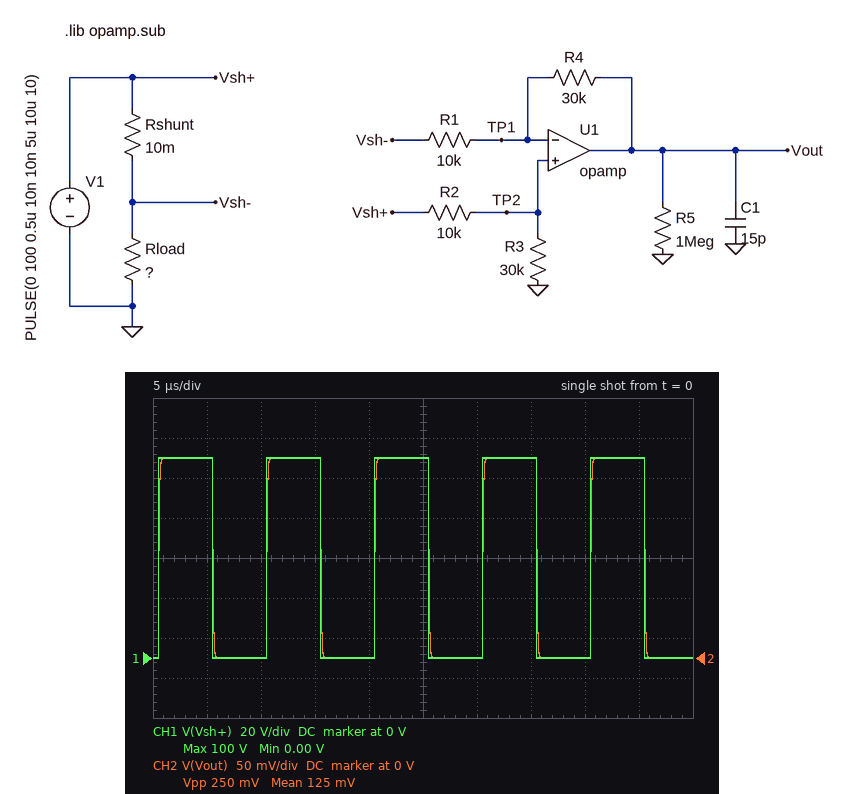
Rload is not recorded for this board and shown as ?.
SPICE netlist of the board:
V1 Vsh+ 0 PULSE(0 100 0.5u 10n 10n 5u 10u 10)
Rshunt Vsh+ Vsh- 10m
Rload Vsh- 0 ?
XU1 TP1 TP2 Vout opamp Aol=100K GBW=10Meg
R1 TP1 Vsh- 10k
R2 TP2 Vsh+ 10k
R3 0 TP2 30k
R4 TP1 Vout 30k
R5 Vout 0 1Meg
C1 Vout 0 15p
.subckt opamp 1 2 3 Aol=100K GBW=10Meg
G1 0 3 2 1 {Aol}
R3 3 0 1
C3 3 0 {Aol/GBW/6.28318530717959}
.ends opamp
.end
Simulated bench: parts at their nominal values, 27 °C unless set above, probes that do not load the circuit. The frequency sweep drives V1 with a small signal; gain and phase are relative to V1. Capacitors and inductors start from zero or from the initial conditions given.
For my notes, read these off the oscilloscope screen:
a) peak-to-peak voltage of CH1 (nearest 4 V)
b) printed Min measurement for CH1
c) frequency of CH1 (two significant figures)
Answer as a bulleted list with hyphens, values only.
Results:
- 100 V
- 0.00 V
- 100 kHz
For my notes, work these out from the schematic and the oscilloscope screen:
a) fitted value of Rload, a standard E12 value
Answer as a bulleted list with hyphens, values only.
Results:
- 12 Ω
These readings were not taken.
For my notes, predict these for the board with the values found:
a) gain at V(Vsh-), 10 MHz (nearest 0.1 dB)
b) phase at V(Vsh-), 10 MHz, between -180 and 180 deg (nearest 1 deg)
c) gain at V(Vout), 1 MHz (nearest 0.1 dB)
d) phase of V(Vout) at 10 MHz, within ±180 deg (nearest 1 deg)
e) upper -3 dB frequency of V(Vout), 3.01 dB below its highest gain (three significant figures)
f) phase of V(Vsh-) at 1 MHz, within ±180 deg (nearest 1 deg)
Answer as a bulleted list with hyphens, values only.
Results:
- 0 dB
- 0 deg
- -52.7 dB
- -76 deg
- 2.50 MHz
- 0 deg
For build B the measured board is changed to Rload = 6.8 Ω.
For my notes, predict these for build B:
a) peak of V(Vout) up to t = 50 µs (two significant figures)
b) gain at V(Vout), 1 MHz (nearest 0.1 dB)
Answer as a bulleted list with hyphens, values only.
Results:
- 440 mV
- -47.8 dB
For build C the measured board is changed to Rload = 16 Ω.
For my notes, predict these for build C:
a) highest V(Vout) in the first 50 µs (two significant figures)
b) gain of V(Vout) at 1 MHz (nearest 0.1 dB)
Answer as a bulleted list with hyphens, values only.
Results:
- 190 mV
- -55.2 dB
